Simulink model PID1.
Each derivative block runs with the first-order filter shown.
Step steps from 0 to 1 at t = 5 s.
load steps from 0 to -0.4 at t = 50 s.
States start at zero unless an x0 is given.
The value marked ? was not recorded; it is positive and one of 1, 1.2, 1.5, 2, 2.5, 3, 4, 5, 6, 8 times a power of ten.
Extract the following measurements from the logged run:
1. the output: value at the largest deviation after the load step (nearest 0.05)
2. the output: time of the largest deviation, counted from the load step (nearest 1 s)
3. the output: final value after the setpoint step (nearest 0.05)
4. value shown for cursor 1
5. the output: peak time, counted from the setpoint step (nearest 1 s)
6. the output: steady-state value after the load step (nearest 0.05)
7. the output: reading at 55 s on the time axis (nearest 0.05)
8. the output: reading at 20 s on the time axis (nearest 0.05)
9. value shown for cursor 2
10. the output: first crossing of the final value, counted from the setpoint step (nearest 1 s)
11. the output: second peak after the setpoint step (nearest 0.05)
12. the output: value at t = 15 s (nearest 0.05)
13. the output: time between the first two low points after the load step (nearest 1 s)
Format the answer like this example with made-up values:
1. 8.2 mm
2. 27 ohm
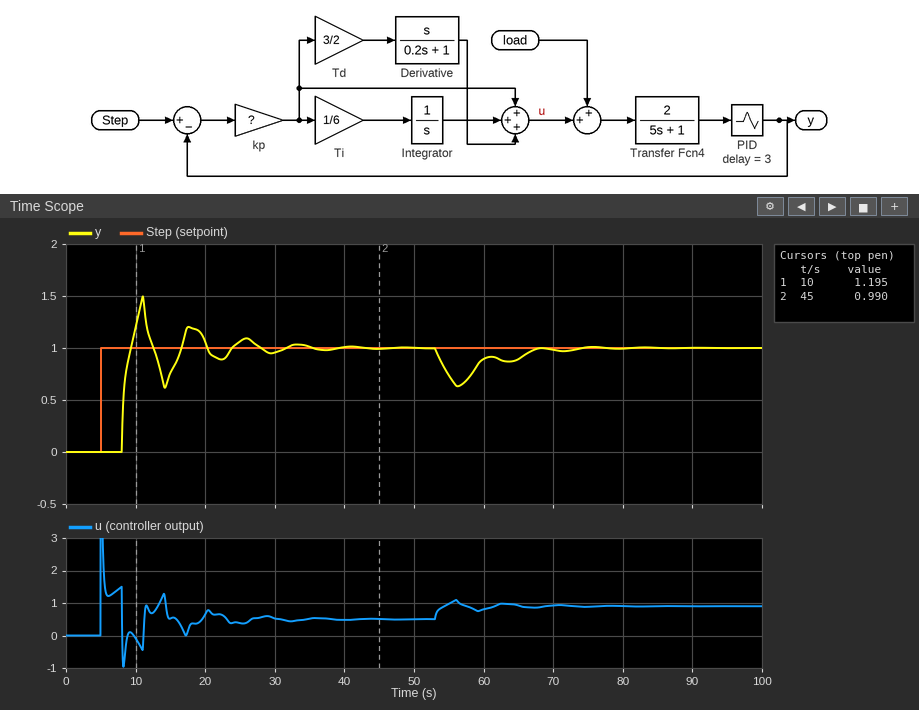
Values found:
1. 0.65
2. 6 s
3. 1.00
4. 1.195
5. 6 s
6. 1.00
7. 0.75
8. 1.05
9. 0.990
10. 4 s
11. 1.20
12. 0.75
13. 7 s
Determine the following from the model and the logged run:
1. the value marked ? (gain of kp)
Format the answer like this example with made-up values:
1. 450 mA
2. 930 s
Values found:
1. 1
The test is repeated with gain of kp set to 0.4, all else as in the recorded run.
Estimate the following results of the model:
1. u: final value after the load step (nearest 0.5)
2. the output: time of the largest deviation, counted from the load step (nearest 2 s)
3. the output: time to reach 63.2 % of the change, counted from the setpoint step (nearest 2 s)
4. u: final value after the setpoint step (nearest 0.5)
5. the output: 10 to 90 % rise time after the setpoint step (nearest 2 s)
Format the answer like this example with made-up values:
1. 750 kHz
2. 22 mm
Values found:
1. 1.0
2. 8 s
3. 8 s
4. 0.5
5. 12 s
